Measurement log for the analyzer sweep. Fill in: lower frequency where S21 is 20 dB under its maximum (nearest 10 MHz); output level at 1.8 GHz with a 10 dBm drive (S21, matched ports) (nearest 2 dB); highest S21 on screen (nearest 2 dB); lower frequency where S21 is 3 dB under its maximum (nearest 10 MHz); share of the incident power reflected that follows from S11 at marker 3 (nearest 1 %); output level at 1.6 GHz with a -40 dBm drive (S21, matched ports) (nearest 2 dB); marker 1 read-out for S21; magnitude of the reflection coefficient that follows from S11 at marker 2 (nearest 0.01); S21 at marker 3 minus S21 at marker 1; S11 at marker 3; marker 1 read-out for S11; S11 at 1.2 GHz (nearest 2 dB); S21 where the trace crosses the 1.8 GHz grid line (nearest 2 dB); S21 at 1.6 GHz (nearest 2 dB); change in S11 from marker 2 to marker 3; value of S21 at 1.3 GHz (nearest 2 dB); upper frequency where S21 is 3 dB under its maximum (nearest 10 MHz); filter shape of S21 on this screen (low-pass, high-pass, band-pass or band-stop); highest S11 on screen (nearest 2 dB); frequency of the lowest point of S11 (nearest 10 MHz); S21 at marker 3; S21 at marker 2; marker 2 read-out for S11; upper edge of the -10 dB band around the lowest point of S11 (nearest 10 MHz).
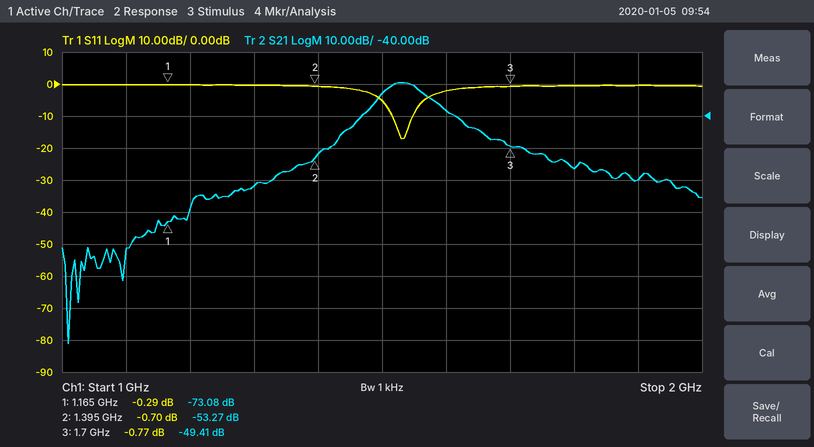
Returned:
1.42 GHz
-46 dBm
-30 dB
1.50 GHz
84 %
-78 dBm
-73.08 dB
0.92
23.67 dB
-0.77 dB
-0.29 dB
0 dB
-56 dB
-38 dB
-0.07 dB
-62 dB
1.56 GHz
band-pass
0 dB
1.53 GHz
-49.41 dB
-53.27 dB
-0.70 dB
1.55 GHz
